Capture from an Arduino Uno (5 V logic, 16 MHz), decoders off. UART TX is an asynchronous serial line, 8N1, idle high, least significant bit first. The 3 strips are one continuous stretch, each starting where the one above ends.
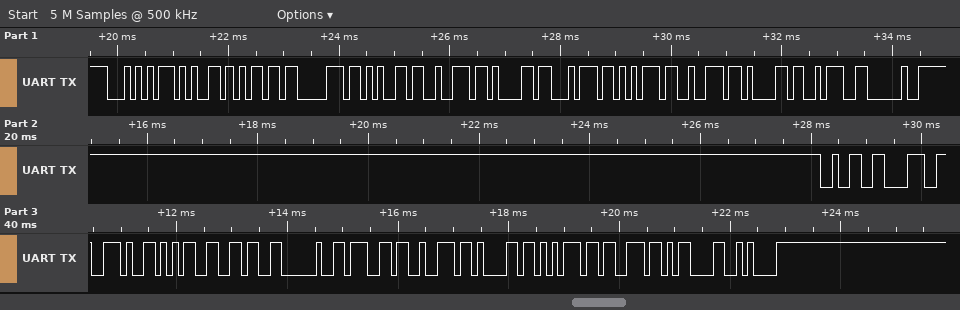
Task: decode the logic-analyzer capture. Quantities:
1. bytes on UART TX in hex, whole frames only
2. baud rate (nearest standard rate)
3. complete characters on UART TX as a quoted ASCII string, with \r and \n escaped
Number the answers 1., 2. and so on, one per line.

1. 54 65 6D 70 65 72 61 74 75 72 61 3A 20 32 38 2E 35 36 20 67 72 61 75 73 0D 0A
2. 9600 baud
3. "Temperatura: 28.56 graus\r\n"
